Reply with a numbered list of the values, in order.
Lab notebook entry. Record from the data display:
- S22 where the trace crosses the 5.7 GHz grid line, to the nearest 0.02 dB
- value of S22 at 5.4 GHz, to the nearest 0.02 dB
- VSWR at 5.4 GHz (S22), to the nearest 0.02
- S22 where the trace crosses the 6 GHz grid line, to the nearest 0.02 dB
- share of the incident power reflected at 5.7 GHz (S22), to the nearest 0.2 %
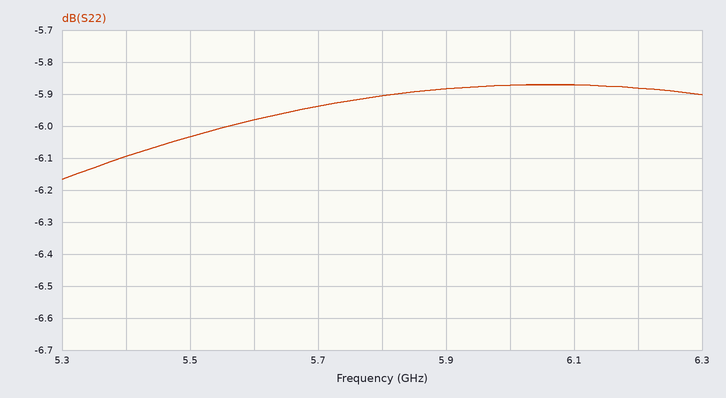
1. -5.94 dB
2. -6.10 dB
3. 2.96
4. -5.88 dB
5. 25.4 %
